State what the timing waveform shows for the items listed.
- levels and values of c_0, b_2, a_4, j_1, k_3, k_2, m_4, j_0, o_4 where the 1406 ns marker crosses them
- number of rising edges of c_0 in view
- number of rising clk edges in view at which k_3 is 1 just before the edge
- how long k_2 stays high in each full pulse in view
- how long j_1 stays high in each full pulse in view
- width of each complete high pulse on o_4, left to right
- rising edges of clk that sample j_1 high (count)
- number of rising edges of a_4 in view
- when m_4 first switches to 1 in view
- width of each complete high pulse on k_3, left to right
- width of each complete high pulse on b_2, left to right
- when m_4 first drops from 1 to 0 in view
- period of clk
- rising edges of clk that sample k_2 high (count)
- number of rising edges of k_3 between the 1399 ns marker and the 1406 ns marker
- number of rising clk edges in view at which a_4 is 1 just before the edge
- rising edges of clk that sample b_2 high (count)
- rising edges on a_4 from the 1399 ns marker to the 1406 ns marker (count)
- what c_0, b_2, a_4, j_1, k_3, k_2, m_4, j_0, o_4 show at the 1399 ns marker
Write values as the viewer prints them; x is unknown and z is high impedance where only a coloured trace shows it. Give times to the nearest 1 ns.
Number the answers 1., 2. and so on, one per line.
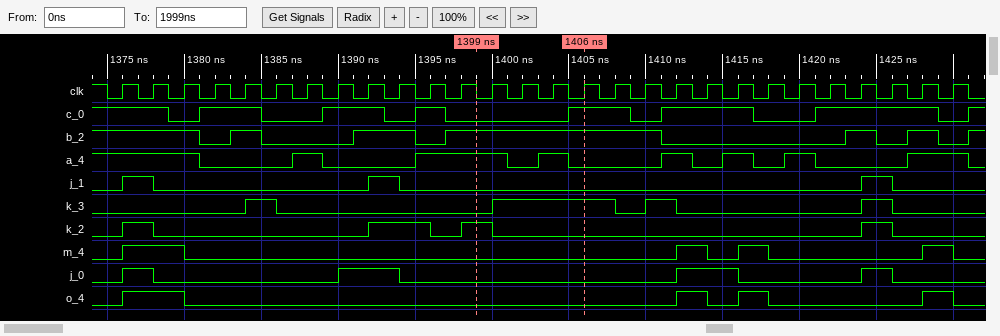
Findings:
1. c_0=1, b_2=1, a_4=0, j_1=0, k_3=1, k_2=0, m_4=0, j_0=0, o_4=0
2. 7
3. 7
4. 2 ns, 4 ns, 2 ns, 2 ns
5. 2 ns, 2 ns, 2 ns
6. 4 ns, 2 ns, 2 ns, 2 ns
7. 3
8. 7
9. 1376 ns
10. 2 ns, 8 ns, 2 ns, 2 ns
11. 2 ns, 4 ns, 14 ns, 2 ns, 2 ns
12. 1380 ns
13. 2 ns
14. 5
15. 1
16. 13
17. 15
18. 1
19. c_0=0, b_2=1, a_4=1, j_1=0, k_3=0, k_2=1, m_4=0, j_0=0, o_4=0
